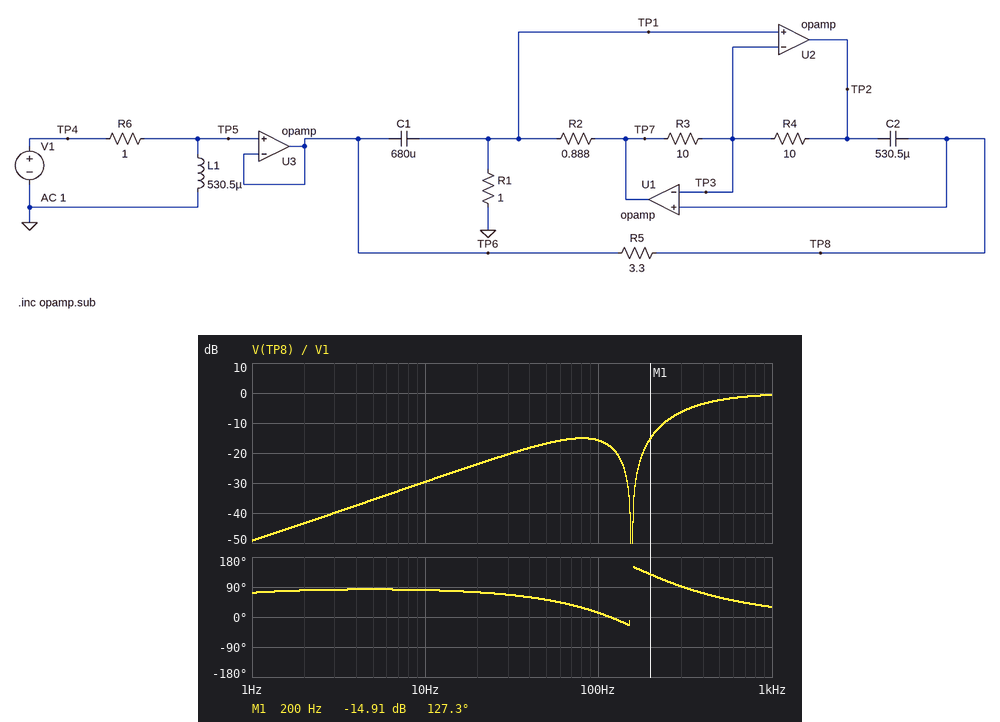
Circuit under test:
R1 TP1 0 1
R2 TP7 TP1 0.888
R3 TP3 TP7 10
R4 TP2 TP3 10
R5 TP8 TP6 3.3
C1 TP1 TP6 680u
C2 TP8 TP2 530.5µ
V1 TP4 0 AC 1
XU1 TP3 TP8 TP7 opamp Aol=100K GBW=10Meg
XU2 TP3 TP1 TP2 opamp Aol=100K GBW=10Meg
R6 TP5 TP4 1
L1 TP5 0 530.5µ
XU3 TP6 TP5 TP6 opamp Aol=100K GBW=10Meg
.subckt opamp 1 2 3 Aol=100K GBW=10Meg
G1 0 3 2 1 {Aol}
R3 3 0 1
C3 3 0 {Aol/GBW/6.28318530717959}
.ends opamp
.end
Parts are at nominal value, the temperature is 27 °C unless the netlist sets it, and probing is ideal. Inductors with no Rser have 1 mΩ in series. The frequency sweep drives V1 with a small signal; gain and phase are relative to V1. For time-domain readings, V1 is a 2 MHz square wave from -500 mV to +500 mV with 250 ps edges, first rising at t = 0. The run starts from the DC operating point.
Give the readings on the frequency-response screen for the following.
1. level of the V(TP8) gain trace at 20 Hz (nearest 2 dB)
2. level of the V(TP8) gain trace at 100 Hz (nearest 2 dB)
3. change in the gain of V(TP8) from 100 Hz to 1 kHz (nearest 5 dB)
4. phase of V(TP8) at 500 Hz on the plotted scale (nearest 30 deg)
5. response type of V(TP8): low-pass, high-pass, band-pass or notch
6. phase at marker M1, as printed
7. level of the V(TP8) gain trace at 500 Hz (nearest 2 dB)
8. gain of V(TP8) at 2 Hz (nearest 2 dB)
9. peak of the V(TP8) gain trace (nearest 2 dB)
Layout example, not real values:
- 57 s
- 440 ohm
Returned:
- -24 dB
- -16 dB
- 15 dB
- 60 deg
- high-pass
- 127.3 deg
- -2 dB
- -44 dB
- 0 dB
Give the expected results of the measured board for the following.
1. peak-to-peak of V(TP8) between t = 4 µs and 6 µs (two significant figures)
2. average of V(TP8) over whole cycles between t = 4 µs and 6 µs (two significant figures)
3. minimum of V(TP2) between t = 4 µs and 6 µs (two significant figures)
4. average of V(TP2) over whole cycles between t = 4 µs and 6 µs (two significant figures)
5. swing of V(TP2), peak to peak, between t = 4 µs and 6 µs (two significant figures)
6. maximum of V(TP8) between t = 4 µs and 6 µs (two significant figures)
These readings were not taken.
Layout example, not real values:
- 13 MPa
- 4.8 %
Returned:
- 1.3 V
- 490 mV
- -150 mV
- 490 mV
- 1.3 V
- 1.1 V
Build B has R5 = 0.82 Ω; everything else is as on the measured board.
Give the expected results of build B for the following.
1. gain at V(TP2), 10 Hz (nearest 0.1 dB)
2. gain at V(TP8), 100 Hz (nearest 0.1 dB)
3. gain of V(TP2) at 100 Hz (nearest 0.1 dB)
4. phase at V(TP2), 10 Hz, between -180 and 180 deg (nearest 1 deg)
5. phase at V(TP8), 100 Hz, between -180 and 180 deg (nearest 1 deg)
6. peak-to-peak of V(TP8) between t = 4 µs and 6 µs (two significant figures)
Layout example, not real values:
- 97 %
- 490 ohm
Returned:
- -48.6 dB
- -10.3 dB
- -51.0 dB
- 85 deg
- 56 deg
- 1.3 V
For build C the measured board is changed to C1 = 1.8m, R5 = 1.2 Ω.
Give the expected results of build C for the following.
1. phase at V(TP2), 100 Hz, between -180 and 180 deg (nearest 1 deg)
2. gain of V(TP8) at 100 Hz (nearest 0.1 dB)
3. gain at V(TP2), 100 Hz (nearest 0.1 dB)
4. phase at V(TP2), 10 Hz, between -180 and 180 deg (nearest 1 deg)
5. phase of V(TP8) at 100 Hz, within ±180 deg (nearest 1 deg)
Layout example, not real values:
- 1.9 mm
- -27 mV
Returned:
- -139 deg
- -11.3 dB
- -17.6 dB
- 84 deg
- 41 deg
